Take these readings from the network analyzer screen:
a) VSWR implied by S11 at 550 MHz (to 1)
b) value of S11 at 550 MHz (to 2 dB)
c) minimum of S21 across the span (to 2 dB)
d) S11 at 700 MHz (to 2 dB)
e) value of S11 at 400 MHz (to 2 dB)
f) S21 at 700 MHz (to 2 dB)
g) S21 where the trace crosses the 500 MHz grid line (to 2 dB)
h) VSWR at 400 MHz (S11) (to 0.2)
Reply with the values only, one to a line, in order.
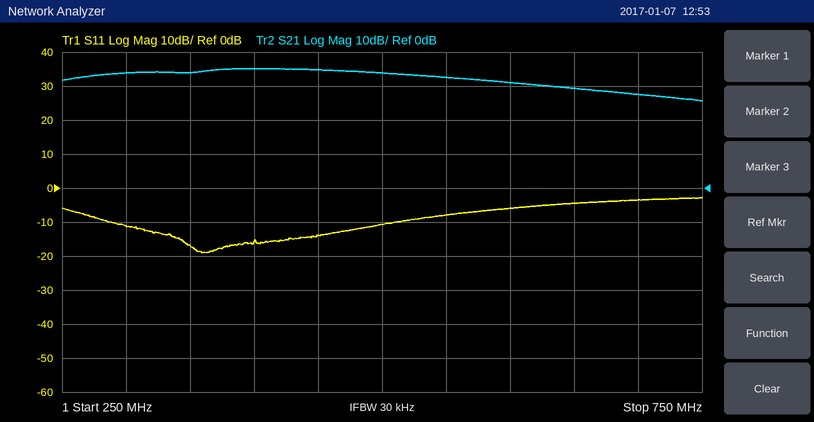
2
-8 dB
26 dB
-4 dB
-16 dB
28 dB
34 dB
1.4
